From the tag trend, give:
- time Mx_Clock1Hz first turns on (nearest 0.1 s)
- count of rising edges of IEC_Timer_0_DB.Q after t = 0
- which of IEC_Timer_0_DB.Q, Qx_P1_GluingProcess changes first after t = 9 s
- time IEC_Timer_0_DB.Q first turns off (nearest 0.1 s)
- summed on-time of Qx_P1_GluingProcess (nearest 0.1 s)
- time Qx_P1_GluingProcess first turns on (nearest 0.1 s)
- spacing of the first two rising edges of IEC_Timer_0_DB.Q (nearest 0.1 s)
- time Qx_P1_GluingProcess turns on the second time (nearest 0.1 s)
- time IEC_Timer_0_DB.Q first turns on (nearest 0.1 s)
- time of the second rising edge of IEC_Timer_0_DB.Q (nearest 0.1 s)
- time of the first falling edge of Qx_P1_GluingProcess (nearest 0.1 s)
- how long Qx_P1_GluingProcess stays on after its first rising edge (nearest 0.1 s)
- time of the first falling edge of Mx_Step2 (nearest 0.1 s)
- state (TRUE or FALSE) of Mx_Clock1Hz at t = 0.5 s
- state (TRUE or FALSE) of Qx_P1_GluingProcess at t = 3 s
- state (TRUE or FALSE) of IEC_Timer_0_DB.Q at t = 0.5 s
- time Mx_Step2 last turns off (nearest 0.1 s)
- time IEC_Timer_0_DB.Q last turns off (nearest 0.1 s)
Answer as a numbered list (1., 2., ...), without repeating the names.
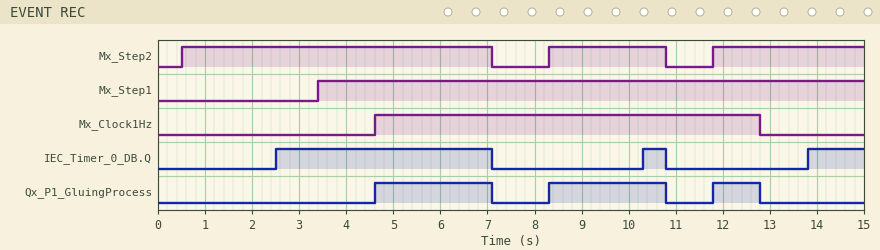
1. 4.6 s
2. 3
3. IEC_Timer_0_DB.Q
4. 7.1 s
5. 6.0 s
6. 4.6 s
7. 7.8 s
8. 8.3 s
9. 2.5 s
10. 10.3 s
11. 7.1 s
12. 2.5 s
13. 7.1 s
14. FALSE
15. FALSE
16. FALSE
17. 10.8 s
18. 10.8 s
